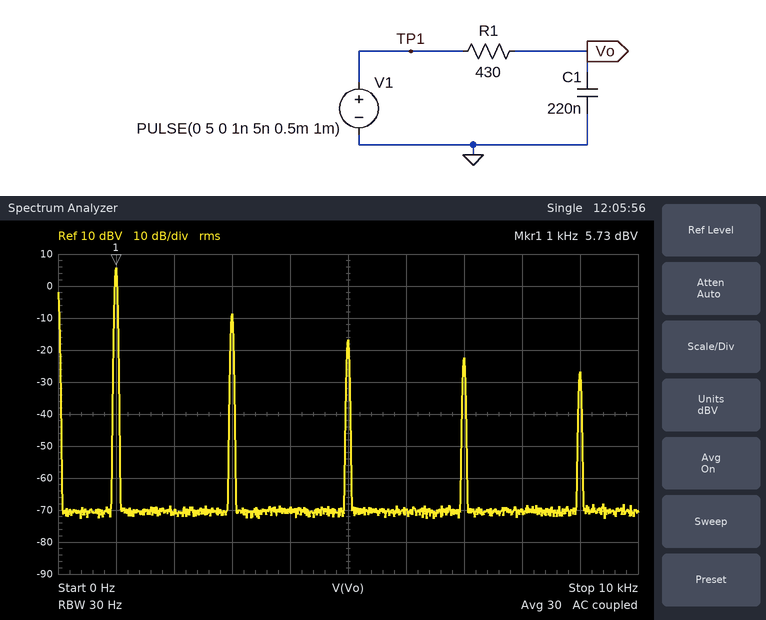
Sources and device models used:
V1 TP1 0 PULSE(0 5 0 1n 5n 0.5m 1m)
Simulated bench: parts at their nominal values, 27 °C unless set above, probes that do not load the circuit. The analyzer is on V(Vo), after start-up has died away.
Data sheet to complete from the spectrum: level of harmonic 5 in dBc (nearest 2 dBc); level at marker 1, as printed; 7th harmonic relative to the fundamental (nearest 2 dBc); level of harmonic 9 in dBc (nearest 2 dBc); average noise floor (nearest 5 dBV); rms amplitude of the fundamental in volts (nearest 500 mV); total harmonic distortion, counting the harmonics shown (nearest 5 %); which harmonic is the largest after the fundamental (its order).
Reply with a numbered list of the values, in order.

1. -22 dBc
2. 5.73 dBV
3. -28 dBc
4. -32 dBc
5. -70 dBV
6. 2.0 V
7. 20 %
8. 3
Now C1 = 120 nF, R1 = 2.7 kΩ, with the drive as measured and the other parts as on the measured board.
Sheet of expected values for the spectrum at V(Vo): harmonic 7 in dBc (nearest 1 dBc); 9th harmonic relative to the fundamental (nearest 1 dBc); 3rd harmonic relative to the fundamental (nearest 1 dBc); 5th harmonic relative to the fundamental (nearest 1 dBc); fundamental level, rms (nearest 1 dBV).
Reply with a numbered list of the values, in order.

1. -33 dBc
2. -37 dBc
3. -18 dBc
4. -27 dBc
5. 0 dBV
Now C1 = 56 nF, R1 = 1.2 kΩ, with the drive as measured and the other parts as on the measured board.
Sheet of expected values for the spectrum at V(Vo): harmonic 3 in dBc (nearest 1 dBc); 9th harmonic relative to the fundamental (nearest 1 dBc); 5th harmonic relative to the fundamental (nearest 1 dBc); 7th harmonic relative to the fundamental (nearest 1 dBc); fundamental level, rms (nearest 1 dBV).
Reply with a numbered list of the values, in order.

1. -13 dBc
2. -30 dBc
3. -21 dBc
4. -26 dBc
5. 6 dBV
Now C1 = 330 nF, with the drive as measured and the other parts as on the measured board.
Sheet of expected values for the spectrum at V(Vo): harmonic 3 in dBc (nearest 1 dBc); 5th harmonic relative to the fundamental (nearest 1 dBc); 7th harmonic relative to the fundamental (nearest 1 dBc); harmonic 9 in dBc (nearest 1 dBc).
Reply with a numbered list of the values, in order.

1. -16 dBc
2. -25 dBc
3. -30 dBc
4. -35 dBc
